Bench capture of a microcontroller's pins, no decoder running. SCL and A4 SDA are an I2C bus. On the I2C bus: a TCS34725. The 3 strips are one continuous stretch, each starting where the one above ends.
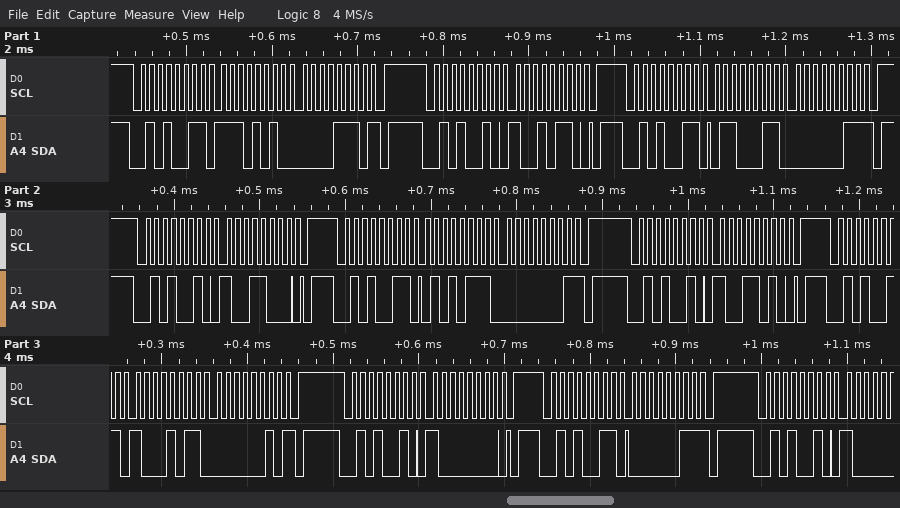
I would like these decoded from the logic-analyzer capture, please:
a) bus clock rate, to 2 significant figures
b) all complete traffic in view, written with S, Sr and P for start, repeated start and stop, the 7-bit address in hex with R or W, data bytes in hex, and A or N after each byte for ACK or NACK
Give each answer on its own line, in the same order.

100 kHz
S 29R A EA A 0E N P S 29W A 96 A P S 29R A 63 A 03 N P S 29W A 98 A P S 29R A 57 A 01 N P S 29W A 9A A P S 29R A 8B A 02 N P S 29W A 80 A P S 29R A 03 N P S 29W A
